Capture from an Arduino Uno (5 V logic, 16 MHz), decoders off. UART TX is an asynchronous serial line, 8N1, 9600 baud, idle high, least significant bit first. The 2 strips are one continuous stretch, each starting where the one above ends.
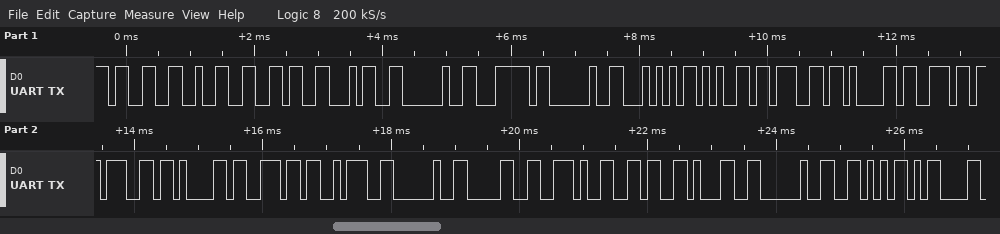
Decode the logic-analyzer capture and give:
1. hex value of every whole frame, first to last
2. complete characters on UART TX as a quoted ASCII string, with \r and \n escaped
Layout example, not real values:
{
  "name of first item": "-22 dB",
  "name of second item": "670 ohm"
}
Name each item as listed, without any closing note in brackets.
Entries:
{
  "hex value of every whole frame, first to last": "33 32 36 34 20 7C 20 54 65 67 61 6E 67 61 6E 3A 20 30 2E 36 31 20 56 0D",
  "complete characters on UART TX as a quoted ASCII string, with \\r and \\n escaped": "\"3264 | Tegangan: 0.61 V\\r\""
}
